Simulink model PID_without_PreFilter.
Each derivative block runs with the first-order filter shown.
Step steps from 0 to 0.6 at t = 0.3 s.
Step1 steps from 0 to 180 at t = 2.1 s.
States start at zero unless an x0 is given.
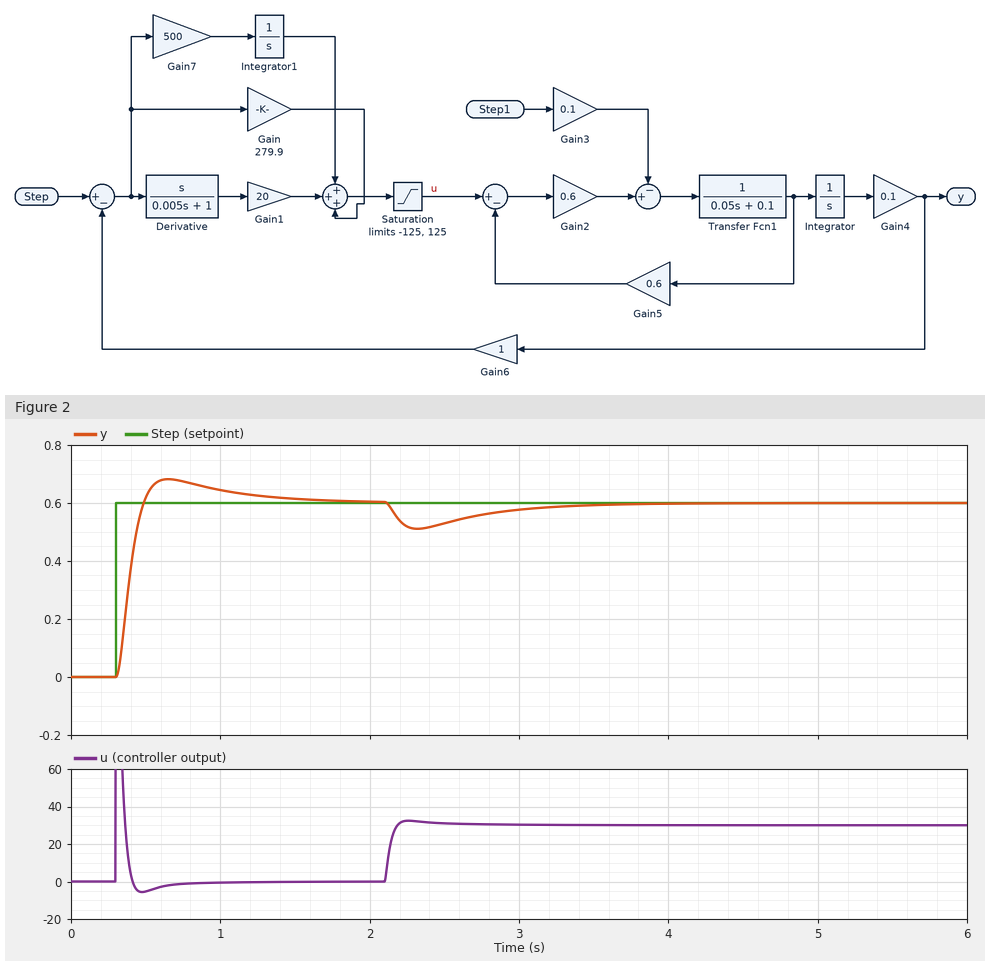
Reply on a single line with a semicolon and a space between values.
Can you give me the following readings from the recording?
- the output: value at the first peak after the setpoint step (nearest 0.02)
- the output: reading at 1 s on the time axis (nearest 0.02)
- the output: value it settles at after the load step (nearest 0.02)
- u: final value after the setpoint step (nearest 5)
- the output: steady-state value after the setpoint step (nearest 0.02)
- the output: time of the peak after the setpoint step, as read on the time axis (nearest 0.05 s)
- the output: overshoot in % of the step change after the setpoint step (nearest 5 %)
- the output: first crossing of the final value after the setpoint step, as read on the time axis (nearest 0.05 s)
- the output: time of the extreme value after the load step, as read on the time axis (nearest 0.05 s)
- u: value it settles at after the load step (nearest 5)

0.68; 0.64; 0.60; 0; 0.60; 0.65 s; 15 %; 0.50 s; 2.30 s; 30
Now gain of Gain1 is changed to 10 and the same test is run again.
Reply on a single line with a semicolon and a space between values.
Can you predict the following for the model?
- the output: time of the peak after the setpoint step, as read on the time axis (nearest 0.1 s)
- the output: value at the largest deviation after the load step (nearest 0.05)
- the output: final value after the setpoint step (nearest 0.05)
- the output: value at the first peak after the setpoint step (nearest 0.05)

0.5 s; 0.50; 0.60; 0.75
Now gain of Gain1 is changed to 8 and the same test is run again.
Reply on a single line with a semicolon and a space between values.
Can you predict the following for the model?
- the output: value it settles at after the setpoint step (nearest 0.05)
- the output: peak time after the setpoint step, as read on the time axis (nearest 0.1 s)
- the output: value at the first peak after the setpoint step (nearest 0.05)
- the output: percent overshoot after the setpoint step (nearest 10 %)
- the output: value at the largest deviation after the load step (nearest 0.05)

0.60; 0.5 s; 0.75; 30 %; 0.50
